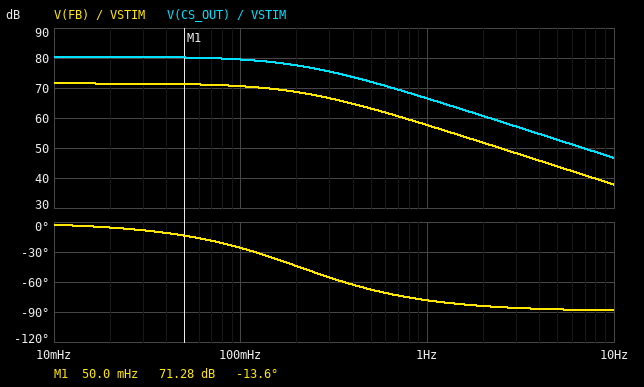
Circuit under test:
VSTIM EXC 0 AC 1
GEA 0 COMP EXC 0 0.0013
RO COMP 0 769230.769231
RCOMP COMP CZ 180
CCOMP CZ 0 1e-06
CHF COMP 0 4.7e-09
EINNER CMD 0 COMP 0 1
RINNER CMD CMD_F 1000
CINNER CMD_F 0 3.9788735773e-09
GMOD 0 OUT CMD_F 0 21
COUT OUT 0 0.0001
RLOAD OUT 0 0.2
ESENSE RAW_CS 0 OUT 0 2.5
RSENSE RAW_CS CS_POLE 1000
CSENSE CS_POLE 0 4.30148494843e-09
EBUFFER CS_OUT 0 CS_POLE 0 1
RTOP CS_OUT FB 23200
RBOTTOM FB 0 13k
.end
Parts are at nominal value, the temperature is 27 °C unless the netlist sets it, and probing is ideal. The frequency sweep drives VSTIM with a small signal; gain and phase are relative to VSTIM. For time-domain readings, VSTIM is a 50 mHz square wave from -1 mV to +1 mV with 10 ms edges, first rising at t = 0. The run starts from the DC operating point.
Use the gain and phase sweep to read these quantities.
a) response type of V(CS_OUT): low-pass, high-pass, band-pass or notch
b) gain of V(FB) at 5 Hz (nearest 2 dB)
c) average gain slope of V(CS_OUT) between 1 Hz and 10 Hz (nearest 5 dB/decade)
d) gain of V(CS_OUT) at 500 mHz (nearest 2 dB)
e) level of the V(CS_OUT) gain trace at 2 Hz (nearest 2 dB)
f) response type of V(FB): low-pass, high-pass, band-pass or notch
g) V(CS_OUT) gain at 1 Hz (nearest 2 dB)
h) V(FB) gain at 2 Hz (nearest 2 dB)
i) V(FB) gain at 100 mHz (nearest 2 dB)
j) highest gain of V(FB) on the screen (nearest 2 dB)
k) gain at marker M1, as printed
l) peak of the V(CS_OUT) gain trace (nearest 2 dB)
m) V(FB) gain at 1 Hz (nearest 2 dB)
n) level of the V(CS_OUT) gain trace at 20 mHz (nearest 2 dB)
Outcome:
low-pass
44 dB
-20 dB/decade
72 dB
60 dB
low-pass
66 dB
52 dB
70 dB
72 dB
71.28 dB
80 dB
58 dB
80 dB
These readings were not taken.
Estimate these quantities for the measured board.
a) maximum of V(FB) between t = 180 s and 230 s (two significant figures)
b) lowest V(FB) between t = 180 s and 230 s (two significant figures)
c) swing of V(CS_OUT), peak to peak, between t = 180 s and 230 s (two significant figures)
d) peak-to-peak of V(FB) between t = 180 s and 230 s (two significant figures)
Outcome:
3.8 V
-3.8 V
21 V
7.5 V
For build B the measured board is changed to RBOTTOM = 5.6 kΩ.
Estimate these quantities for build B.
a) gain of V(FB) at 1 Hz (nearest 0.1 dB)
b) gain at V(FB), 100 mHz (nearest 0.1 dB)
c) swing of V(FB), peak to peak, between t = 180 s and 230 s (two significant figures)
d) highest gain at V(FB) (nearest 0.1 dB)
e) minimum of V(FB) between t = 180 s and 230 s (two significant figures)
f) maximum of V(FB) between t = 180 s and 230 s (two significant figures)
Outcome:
52.3 dB
65.3 dB
4.1 V
66.2 dB
-2.0 V
2.0 V
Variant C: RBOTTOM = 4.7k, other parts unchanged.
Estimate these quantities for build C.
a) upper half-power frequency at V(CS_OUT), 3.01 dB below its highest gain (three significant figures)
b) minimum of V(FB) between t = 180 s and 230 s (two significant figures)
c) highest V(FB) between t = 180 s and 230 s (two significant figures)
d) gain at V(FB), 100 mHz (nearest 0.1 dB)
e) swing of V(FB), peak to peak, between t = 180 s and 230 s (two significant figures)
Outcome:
206 mHz
-1.8 V
1.8 V
64.0 dB
3.5 V
